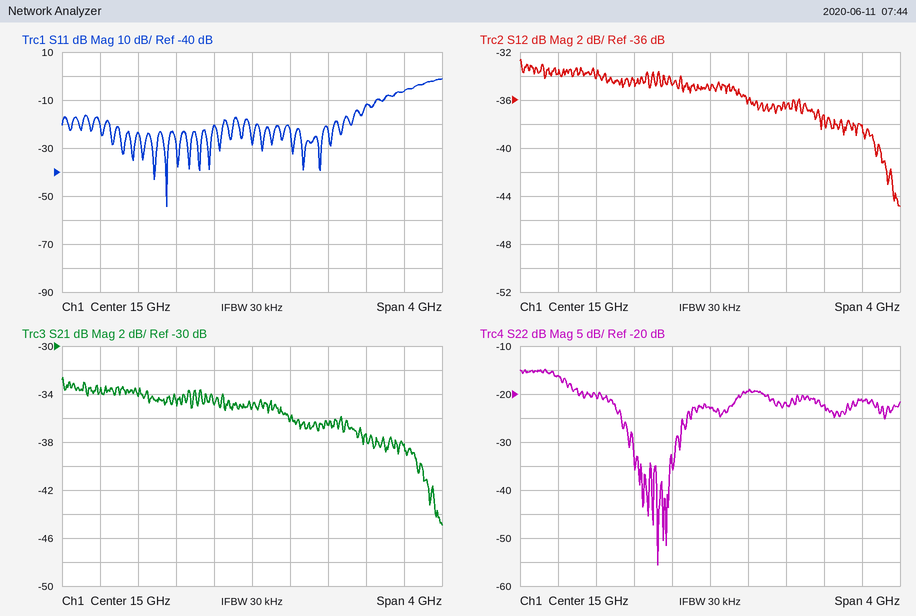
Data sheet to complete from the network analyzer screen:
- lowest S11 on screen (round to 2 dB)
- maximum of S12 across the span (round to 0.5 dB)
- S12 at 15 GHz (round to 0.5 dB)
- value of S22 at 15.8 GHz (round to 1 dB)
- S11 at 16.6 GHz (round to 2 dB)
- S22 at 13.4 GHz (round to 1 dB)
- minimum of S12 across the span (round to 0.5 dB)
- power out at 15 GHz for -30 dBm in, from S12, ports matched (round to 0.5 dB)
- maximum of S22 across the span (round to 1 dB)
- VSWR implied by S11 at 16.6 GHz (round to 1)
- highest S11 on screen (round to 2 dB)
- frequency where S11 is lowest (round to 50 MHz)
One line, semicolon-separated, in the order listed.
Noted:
-54 dB; -32.5 dB; -35.0 dB; -22 dB; -6 dB; -16 dB; -45.0 dB; -65.0 dBm; -15 dB; 3; -2 dB; 14.10 GHz
